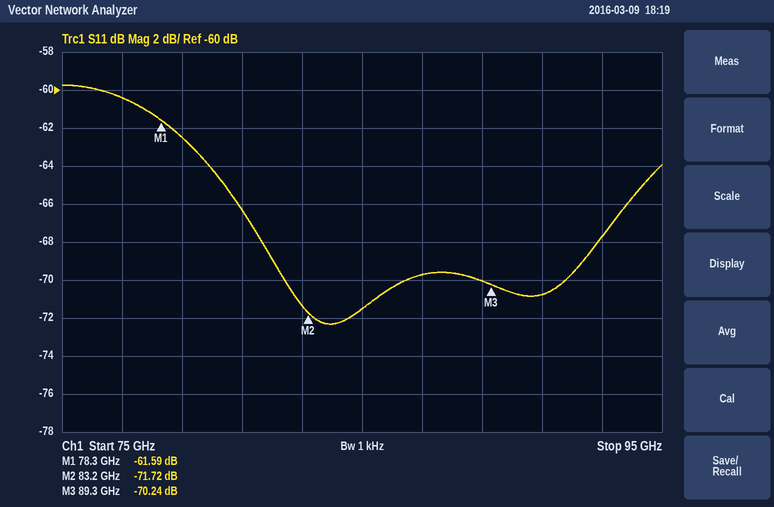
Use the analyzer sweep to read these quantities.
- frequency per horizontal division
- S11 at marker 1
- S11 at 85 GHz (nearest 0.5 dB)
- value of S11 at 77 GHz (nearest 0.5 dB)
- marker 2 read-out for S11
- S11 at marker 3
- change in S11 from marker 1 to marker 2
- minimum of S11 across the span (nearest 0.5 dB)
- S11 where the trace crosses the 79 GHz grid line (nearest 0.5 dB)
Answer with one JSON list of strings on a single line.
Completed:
["2 GHz", "-61.59 dB", "-71.5 dB", "-60.5 dB", "-71.72 dB", "-70.24 dB", "-10.13 dB", "-72.5 dB", "-62.5 dB"]
